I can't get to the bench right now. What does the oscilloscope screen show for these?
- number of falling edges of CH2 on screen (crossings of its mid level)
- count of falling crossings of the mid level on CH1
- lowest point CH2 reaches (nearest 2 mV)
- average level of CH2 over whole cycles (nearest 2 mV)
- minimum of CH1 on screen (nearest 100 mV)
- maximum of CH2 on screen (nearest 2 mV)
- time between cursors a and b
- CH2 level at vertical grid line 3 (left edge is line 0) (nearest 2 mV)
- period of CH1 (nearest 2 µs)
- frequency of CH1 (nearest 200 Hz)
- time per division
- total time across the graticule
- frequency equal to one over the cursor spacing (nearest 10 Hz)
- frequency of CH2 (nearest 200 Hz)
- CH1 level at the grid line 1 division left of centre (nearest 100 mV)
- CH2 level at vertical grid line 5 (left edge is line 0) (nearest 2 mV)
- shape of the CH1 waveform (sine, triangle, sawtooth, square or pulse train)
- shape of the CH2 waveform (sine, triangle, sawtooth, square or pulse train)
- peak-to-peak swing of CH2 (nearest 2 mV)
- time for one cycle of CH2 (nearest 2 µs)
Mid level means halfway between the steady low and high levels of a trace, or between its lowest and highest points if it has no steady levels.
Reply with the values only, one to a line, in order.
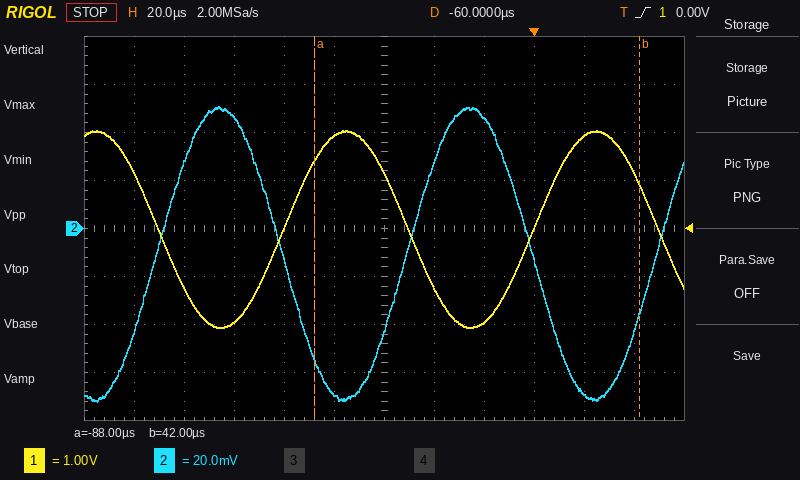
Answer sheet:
2
3
-72 mV
-10 mV
-2.1 V
50 mV
130 µs
46 mV
100 µs
10.0 kHz
20 µs
240 µs
7.69 kHz
10.0 kHz
1.9 V
-68 mV
sine
sine
122 mV
100 µs
